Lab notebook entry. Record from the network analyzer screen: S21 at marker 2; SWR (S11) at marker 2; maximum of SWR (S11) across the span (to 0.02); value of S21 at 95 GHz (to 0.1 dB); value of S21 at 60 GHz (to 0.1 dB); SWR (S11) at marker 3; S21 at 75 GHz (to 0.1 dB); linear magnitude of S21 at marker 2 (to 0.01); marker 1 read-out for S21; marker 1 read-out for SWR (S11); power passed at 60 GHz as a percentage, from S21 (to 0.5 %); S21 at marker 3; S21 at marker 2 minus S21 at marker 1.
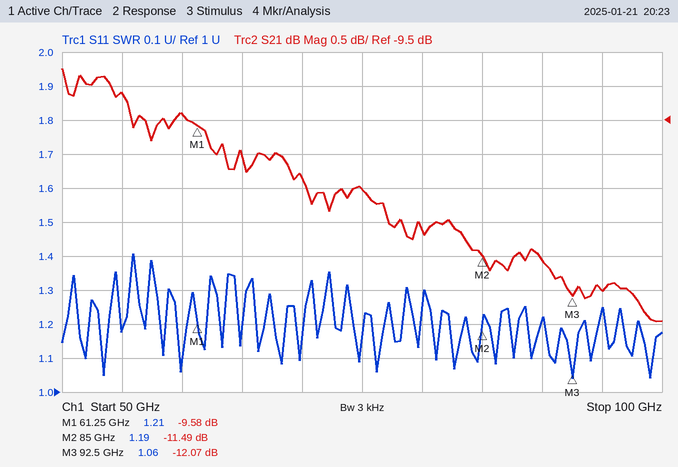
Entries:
-11.49 dB
1.19
1.40
-12.0 dB
-9.4 dB
1.06
-10.5 dB
0.27
-9.58 dB
1.21
11.5 %
-12.07 dB
-1.91 dB
